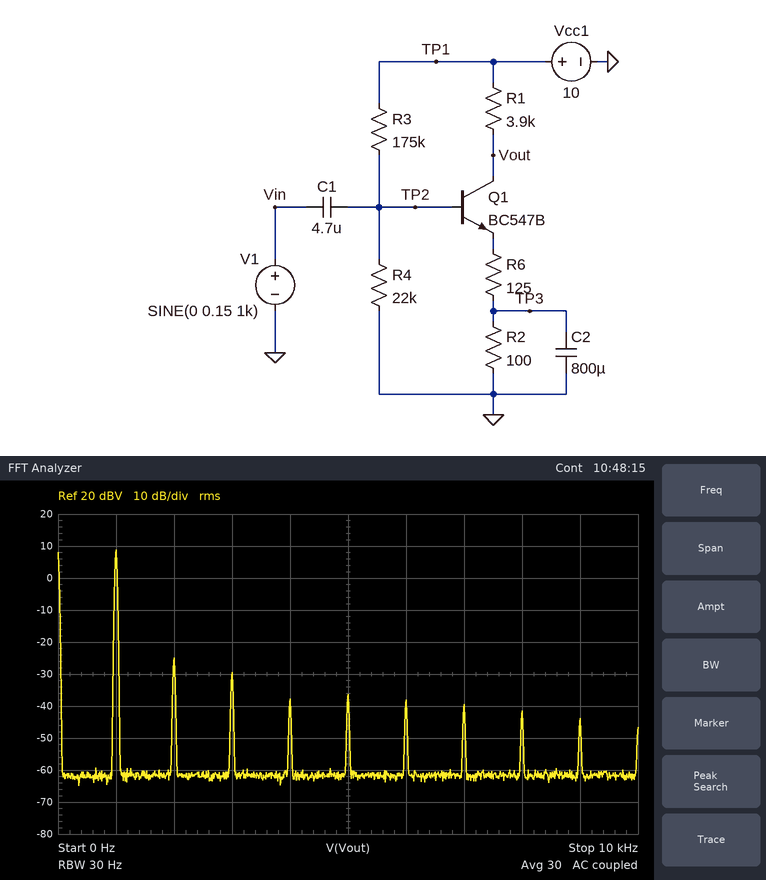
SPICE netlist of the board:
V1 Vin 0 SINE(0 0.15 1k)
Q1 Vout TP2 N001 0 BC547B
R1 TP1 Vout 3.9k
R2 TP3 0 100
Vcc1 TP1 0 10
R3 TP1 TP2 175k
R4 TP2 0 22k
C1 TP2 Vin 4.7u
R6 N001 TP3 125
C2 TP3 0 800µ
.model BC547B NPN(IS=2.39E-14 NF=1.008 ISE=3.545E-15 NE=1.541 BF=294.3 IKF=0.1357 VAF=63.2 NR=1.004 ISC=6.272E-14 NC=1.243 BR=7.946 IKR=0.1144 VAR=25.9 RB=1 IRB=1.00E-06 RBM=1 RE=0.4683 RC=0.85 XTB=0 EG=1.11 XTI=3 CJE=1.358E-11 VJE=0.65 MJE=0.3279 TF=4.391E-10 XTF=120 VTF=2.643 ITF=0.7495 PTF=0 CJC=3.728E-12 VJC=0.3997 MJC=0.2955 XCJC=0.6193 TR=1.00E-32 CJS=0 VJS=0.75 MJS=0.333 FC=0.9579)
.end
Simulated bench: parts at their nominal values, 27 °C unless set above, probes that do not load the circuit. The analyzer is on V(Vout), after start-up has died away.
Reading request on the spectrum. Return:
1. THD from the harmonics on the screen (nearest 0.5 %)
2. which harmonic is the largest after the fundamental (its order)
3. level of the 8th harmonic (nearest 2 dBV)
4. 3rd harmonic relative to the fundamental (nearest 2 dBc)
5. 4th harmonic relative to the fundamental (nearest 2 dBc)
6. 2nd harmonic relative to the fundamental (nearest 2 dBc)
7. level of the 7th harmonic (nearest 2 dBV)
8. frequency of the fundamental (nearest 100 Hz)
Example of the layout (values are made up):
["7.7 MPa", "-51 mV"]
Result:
["2.5 %", "2", "-42 dBV", "-38 dBc", "-46 dBc", "-34 dBc", "-40 dBV", "1.0 kHz"]
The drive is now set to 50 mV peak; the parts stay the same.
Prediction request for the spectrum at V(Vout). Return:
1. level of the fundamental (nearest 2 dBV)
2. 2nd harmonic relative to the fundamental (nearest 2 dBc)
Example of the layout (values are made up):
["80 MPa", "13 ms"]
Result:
["0 dBV", "-44 dBc"]
